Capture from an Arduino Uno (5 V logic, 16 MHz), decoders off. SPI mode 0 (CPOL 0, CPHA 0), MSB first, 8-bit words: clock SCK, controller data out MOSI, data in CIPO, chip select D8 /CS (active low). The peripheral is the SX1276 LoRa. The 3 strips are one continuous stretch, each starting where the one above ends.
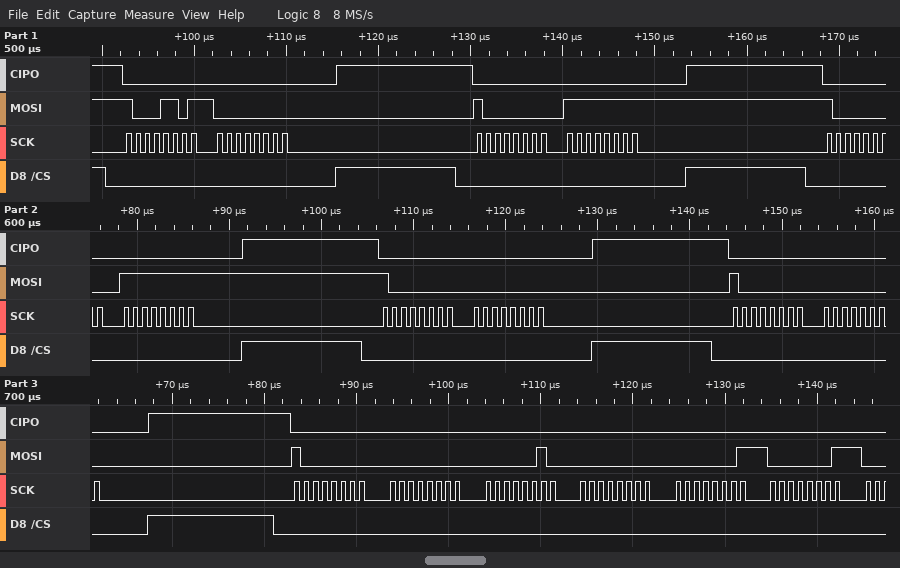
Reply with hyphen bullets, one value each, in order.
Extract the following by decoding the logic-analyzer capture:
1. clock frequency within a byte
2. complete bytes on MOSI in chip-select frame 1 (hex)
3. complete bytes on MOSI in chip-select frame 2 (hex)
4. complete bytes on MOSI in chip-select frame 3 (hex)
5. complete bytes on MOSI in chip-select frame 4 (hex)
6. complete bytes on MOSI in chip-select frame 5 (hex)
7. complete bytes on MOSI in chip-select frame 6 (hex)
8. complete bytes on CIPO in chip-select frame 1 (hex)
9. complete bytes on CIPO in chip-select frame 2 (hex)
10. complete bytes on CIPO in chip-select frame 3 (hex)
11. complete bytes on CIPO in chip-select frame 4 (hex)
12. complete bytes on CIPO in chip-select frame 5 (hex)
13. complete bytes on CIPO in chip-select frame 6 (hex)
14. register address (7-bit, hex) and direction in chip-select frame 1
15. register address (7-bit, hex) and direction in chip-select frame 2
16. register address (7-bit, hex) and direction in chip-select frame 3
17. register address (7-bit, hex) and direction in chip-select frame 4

- 1 MHz
- 8D 00
- 80 FF
- 80 FF
- 80 00
- 80 00
- 80 00 02 00 01 01
- 00 00
- 00 00
- 00 00
- 00 00
- 00 00
- 00 00 00 00 00 00
- 0x0D write
- 0x00 write
- 0x00 write
- 0x00 write
